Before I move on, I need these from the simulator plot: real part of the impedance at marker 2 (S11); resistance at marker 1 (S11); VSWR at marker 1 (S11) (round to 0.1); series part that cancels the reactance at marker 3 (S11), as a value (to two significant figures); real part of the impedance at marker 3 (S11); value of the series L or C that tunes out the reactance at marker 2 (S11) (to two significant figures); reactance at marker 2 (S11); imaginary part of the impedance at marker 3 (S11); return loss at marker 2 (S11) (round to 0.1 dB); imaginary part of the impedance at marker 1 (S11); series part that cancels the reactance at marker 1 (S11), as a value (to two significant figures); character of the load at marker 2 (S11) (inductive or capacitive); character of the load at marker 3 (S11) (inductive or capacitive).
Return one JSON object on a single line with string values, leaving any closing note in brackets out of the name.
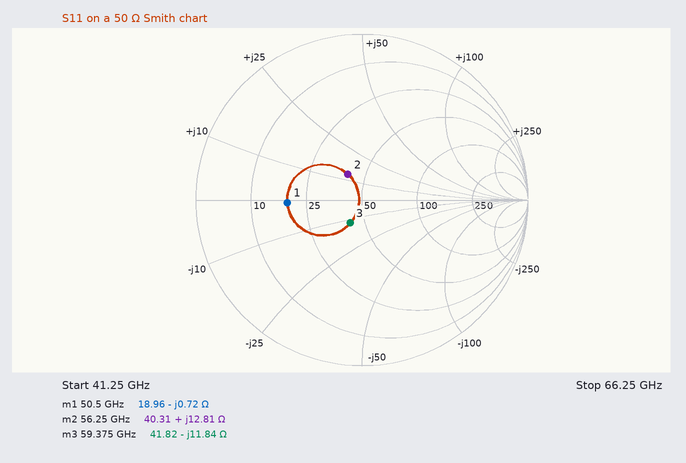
{"real part of the impedance at marker 2": "40.31 Ω", "resistance at marker 1": "18.96 Ω", "VSWR at marker 1 (S11)": "2.6", "series part that cancels the reactance at marker 3 (S11), as a value": "32 pH", "real part of the impedance at marker 3": "41.82 Ω", "value of the series L or C that tunes out the reactance at marker 2 (S11)": "220 fF", "reactance at marker 2": "+12.81 Ω", "imaginary part of the impedance at marker 3": "-11.84 Ω", "return loss at marker 2 (S11)": "15.1 dB", "imaginary part of the impedance at marker 1": "-0.72 Ω", "series part that cancels the reactance at marker 1 (S11), as a value": "2.3 pH", "character of the load at marker 2 (S11)": "inductive", "character of the load at marker 3 (S11)": "capacitive"}
